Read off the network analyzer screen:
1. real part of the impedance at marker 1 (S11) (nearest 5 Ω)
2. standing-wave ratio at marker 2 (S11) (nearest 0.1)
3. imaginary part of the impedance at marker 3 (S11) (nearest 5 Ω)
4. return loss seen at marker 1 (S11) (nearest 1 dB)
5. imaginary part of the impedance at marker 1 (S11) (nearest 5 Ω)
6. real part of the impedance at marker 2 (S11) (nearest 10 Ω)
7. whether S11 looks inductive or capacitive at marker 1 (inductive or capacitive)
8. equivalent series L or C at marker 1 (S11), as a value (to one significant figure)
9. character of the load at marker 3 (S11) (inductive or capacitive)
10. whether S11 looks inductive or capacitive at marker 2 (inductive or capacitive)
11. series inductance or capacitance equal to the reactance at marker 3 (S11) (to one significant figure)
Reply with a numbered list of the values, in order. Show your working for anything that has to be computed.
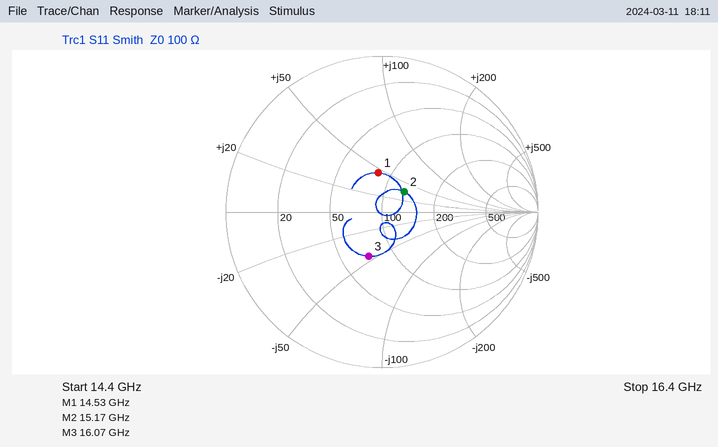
1. 85 Ω
2. 1.5
3. -45 Ω
4. 12 dB
5. +45 Ω
6. 130 Ω
7. inductive
8. L = 45 Ω/(2π × 14.53 GHz) ≈ 493 pH, so 500 pH to one significant figure
9. capacitive
10. inductive
11. C = 1/(2π × 16.07 GHz × 45 Ω) ≈ 220 fF, so 200 fF to one significant figure
